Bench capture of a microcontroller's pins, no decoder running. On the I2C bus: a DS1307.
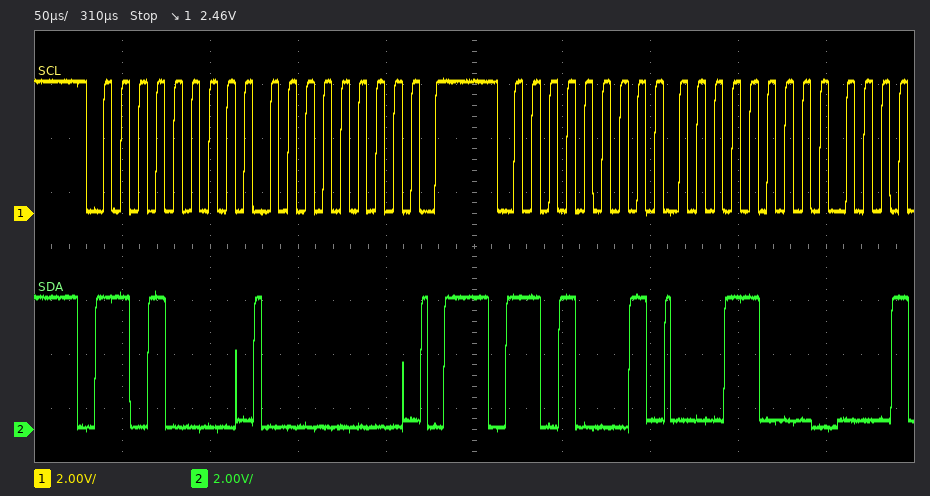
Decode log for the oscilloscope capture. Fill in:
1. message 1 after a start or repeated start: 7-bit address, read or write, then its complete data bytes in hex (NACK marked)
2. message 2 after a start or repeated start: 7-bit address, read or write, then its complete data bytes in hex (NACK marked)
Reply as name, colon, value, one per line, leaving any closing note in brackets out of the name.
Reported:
message 1 after a start or repeated start: 7-bit address, read or write, then its complete data bytes in hex: 0x68 write: 00
message 2 after a start or repeated start: 7-bit address, read or write, then its complete data bytes in hex: 0x68 read: 18
